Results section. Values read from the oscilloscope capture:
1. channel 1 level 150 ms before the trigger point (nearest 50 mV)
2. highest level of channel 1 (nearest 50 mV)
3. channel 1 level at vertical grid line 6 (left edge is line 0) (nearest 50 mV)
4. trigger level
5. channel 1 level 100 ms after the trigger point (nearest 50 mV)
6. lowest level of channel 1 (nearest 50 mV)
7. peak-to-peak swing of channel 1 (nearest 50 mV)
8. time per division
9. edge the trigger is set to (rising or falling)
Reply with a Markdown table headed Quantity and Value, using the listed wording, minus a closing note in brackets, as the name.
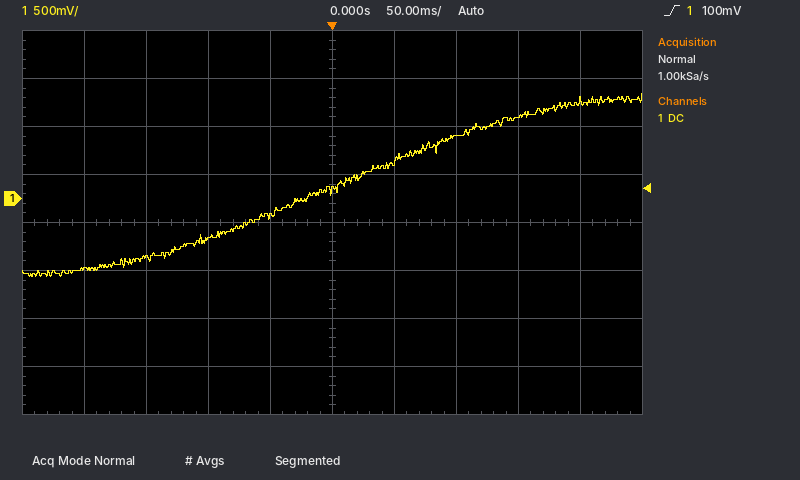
| Quantity | Value |
|---|---|
| channel 1 level 150 ms before the trigger point | -600 mV |
| highest level of channel 1 | 1.10 V |
| channel 1 level at vertical grid line 6 (left edge is line 0) | 400 mV |
| trigger level | 100 mV |
| channel 1 level 100 ms after the trigger point | 650 mV |
| lowest level of channel 1 | -800 mV |
| peak-to-peak swing of channel 1 | 1.90 V |
| time per division | 50 ms |
| edge the trigger is set to | rising |
